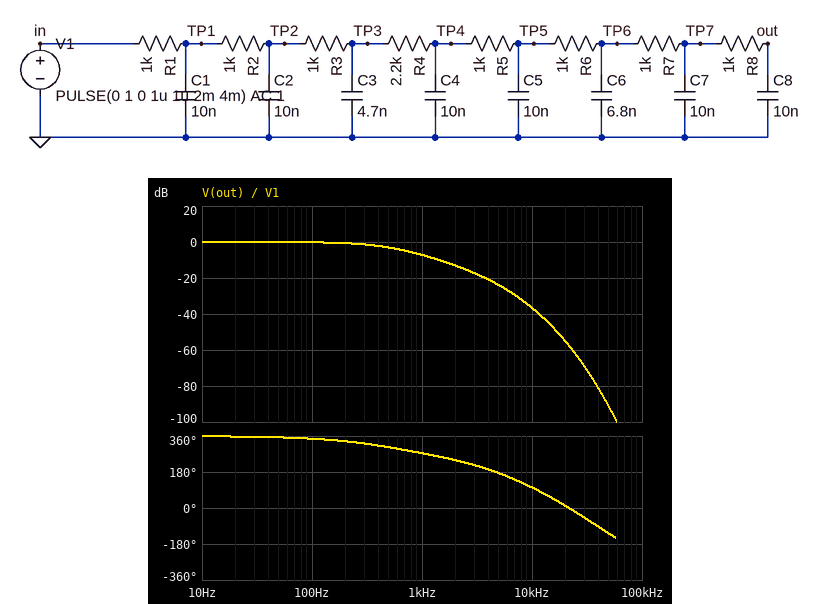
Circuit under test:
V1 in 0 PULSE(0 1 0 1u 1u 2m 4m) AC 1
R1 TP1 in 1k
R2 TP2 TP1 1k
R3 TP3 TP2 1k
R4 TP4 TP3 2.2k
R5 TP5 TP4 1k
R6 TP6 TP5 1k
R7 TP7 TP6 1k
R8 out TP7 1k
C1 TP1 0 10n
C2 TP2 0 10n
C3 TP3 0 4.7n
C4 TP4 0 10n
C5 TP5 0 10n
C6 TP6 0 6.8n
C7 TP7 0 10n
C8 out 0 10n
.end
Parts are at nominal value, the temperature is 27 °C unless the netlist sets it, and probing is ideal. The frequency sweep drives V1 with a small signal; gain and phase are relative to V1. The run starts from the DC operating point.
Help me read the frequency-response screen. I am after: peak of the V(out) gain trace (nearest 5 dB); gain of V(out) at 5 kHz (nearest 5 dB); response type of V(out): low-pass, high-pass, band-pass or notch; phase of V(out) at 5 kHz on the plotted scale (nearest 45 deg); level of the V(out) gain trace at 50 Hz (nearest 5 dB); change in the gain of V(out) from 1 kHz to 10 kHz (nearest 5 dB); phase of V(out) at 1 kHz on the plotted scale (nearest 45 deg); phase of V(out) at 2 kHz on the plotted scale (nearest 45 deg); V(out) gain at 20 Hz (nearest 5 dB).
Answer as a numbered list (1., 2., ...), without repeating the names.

1. 0 dB
2. -25 dB
3. low-pass
4. 180 deg
5. 0 dB
6. -30 dB
7. 270 deg
8. 225 deg
9. 0 dB
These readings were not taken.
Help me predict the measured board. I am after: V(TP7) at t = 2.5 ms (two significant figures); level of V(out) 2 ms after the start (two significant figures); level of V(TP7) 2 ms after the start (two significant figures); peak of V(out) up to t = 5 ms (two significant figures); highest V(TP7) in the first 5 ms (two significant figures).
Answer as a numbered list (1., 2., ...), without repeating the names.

1. 250 mV
2. 1.0 V
3. 1.0 V
4. 1.0 V
5. 1.0 V
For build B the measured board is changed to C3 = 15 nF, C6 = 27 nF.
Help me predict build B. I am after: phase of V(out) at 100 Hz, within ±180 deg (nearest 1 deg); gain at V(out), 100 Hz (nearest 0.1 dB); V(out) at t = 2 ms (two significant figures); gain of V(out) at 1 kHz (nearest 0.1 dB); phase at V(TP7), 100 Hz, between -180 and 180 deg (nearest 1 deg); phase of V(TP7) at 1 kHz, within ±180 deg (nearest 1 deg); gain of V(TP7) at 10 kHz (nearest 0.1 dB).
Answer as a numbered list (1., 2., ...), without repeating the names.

1. -20 deg
2. -0.4 dB
3. 980 mV
4. -10.3 dB
5. -19 deg
6. -98 deg
7. -43.0 dB
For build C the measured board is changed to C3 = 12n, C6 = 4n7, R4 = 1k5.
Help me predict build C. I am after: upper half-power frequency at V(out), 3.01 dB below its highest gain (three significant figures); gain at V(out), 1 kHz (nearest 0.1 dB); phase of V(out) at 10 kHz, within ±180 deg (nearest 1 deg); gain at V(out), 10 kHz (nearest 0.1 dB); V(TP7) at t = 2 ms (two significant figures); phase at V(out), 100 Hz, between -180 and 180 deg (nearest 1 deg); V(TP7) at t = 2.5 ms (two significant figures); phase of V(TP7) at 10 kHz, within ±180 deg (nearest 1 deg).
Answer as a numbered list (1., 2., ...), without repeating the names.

1. 543 Hz
2. -6.6 dB
3. 98 deg
4. -36.8 dB
5. 1.0 V
6. -13 deg
7. 220 mV
8. 130 deg
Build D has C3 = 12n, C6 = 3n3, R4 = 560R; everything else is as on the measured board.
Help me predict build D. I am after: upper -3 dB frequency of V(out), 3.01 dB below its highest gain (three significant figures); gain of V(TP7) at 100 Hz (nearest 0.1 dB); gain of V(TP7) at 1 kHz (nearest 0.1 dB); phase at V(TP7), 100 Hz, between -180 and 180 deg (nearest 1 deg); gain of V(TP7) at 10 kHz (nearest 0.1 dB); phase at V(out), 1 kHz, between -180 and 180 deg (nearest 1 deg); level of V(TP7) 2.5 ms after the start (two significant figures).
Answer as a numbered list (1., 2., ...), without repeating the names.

1. 636 Hz
2. -0.1 dB
3. -5.5 dB
4. -11 deg
5. -32.5 dB
6. -79 deg
7. 160 mV
